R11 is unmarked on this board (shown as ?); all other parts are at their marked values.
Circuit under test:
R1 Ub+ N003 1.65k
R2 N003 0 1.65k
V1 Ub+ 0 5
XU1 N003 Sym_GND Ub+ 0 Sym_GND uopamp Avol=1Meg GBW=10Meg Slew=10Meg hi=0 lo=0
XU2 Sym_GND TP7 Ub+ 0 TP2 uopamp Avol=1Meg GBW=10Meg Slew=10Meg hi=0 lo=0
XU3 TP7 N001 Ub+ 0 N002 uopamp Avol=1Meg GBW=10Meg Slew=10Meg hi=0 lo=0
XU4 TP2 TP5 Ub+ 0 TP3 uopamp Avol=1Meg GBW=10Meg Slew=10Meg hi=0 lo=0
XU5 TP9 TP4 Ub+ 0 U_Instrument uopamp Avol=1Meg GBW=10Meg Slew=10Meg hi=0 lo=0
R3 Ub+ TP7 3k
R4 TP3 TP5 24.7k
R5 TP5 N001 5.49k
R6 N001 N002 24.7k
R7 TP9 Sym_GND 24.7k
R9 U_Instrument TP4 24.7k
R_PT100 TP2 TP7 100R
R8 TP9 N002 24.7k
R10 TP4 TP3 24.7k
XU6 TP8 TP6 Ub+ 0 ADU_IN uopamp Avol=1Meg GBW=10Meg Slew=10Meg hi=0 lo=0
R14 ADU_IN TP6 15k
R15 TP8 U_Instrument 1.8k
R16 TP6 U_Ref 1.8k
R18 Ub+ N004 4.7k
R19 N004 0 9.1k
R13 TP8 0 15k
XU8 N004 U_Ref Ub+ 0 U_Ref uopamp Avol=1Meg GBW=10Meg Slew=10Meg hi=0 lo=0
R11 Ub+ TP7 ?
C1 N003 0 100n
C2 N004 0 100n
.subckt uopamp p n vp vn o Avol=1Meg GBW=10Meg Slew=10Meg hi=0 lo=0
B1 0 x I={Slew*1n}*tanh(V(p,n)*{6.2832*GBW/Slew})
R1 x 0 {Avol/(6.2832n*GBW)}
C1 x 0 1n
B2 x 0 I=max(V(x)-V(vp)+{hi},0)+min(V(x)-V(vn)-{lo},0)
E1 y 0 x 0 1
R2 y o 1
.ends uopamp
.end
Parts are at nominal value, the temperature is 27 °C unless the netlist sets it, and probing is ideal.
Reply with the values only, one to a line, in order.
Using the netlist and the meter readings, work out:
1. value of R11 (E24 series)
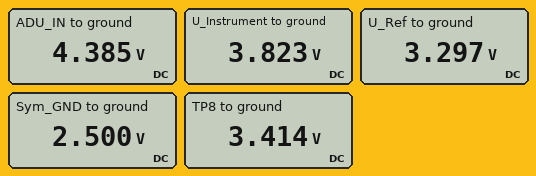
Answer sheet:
5.1 kΩ
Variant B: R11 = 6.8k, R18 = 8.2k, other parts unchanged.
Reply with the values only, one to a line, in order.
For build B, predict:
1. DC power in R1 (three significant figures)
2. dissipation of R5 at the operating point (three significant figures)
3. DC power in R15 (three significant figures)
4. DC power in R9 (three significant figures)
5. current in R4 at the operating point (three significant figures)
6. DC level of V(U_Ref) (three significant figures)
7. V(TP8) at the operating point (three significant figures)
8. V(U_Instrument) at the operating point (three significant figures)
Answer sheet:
3.79 mW
2.63 µW
87.3 µW
35.1 µW
21.9 µA
2.63 V
3.30 V
3.70 V
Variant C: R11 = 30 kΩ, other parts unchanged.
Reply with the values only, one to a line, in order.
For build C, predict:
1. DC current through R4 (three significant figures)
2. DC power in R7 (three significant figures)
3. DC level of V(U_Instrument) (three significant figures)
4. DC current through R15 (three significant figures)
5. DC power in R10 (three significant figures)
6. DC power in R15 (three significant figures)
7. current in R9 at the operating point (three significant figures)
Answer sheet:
16.7 µA
1.72 µW
3.42 V
203 µA
20.4 µW
74.4 µW
28.8 µA
